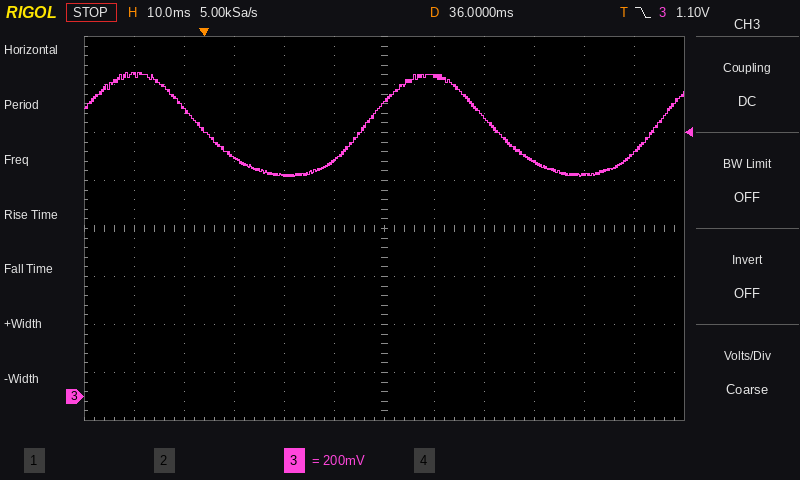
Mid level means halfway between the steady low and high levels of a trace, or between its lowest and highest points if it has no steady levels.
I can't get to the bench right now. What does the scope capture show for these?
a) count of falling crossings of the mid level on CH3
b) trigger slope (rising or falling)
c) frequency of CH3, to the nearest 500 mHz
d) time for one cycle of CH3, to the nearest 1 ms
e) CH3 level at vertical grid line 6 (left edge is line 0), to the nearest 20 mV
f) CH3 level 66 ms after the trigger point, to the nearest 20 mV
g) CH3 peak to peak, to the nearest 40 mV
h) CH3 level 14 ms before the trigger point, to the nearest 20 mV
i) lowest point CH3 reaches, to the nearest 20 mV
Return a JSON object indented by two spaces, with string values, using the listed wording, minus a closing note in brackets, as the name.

{
  "count of falling crossings of the mid level on CH3": "2",
  "trigger slope": "falling",
  "frequency of CH3, to the nearest 500 mHz": "17.0 Hz",
  "time for one cycle of CH3, to the nearest 1 ms": "58 ms",
  "CH3 level at vertical grid line 6 (left edge is line 0), to the nearest 20 mV": "1.22 V",
  "CH3 level 66 ms after the trigger point, to the nearest 20 mV": "980 mV",
  "CH3 peak to peak, to the nearest 40 mV": "440 mV",
  "CH3 level 14 ms before the trigger point, to the nearest 20 mV": "1.34 V",
  "lowest point CH3 reaches, to the nearest 20 mV": "920 mV"
}
